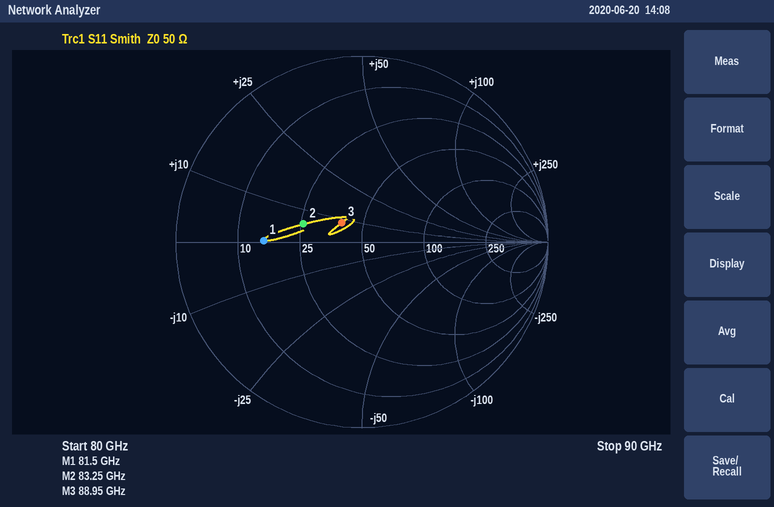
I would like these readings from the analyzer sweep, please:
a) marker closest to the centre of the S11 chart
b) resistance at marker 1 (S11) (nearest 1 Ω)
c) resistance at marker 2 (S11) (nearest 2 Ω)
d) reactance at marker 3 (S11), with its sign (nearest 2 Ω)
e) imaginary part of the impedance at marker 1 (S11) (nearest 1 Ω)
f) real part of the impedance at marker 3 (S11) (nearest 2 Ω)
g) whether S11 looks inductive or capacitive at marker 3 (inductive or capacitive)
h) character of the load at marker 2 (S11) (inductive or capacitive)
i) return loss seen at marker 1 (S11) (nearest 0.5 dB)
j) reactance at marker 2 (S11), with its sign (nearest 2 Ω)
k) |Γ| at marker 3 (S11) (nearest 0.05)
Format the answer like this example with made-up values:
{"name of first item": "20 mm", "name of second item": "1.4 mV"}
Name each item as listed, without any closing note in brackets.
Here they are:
{"marker closest to the centre of the S11 chart": "marker 3", "resistance at marker 1 (S11)": "15 Ω", "resistance at marker 2 (S11)": "26 Ω", "reactance at marker 3 (S11), with its sign": "+8 Ω", "imaginary part of the impedance at marker 1 (S11)": "0 Ω", "real part of the impedance at marker 3 (S11)": "40 Ω", "whether S11 looks inductive or capacitive at marker 3": "inductive", "character of the load at marker 2 (S11)": "inductive", "return loss seen at marker 1 (S11)": "5.5 dB", "reactance at marker 2 (S11), with its sign": "+6 Ω", "|Γ| at marker 3 (S11)": "0.15"}
